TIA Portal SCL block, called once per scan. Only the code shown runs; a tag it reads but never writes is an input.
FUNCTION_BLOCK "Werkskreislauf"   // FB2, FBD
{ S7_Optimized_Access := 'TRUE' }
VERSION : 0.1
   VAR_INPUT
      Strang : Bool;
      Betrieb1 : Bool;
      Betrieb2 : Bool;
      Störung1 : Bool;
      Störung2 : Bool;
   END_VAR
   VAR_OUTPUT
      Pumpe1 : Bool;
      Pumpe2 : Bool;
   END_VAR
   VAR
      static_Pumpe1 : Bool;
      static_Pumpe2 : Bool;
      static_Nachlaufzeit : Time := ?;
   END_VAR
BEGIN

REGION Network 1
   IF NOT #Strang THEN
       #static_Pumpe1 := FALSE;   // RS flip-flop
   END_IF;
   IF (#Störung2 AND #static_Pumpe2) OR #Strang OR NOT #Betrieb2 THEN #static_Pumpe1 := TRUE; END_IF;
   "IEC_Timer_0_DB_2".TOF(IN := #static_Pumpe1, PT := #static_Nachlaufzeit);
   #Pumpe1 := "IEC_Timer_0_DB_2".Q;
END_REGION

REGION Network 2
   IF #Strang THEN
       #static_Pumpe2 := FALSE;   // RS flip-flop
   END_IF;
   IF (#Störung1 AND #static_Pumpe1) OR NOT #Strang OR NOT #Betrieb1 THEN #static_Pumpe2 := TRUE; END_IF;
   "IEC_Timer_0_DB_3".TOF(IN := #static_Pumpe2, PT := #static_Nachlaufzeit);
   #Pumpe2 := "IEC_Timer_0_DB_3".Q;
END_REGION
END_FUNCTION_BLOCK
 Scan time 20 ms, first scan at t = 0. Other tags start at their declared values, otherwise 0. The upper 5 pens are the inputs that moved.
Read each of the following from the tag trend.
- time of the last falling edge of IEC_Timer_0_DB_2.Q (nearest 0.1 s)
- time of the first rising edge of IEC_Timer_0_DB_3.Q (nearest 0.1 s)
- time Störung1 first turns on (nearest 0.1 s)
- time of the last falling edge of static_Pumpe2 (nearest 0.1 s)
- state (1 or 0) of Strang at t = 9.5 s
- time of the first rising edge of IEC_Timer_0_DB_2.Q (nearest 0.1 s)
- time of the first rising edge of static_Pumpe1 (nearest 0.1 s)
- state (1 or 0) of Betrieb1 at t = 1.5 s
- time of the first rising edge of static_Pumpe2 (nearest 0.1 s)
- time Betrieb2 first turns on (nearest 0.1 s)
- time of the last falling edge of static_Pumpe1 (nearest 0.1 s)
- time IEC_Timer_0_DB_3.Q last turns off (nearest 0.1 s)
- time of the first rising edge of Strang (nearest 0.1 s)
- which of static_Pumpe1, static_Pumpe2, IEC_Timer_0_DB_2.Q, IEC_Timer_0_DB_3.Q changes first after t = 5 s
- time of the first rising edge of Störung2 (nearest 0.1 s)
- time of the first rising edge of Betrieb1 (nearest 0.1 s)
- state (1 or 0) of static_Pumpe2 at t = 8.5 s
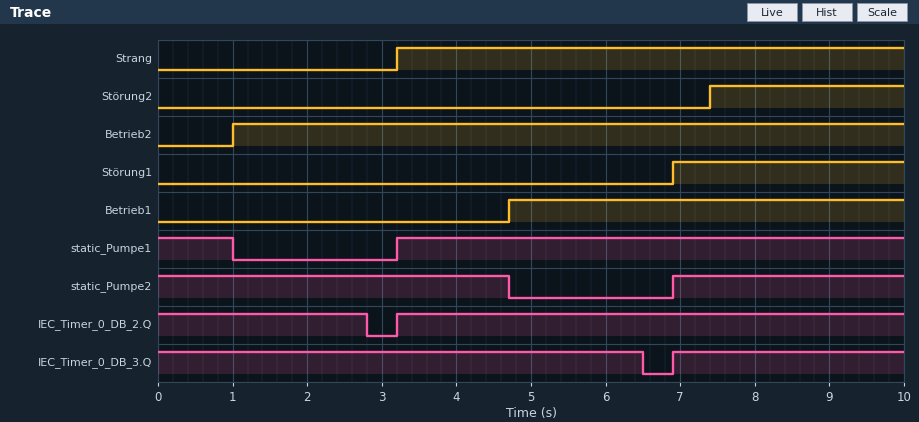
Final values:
2.8 s
6.9 s
6.9 s
4.7 s
1
3.2 s
3.2 s
0
6.9 s
1.0 s
1.0 s
6.5 s
3.2 s
IEC_Timer_0_DB_3.Q
7.4 s
4.7 s
1
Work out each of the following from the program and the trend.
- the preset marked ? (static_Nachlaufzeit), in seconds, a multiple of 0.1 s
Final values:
1.8 s
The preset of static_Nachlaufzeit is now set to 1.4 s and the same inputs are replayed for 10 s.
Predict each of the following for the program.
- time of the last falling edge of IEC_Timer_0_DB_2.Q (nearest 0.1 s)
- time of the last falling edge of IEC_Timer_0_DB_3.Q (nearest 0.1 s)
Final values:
2.4 s
6.1 s
